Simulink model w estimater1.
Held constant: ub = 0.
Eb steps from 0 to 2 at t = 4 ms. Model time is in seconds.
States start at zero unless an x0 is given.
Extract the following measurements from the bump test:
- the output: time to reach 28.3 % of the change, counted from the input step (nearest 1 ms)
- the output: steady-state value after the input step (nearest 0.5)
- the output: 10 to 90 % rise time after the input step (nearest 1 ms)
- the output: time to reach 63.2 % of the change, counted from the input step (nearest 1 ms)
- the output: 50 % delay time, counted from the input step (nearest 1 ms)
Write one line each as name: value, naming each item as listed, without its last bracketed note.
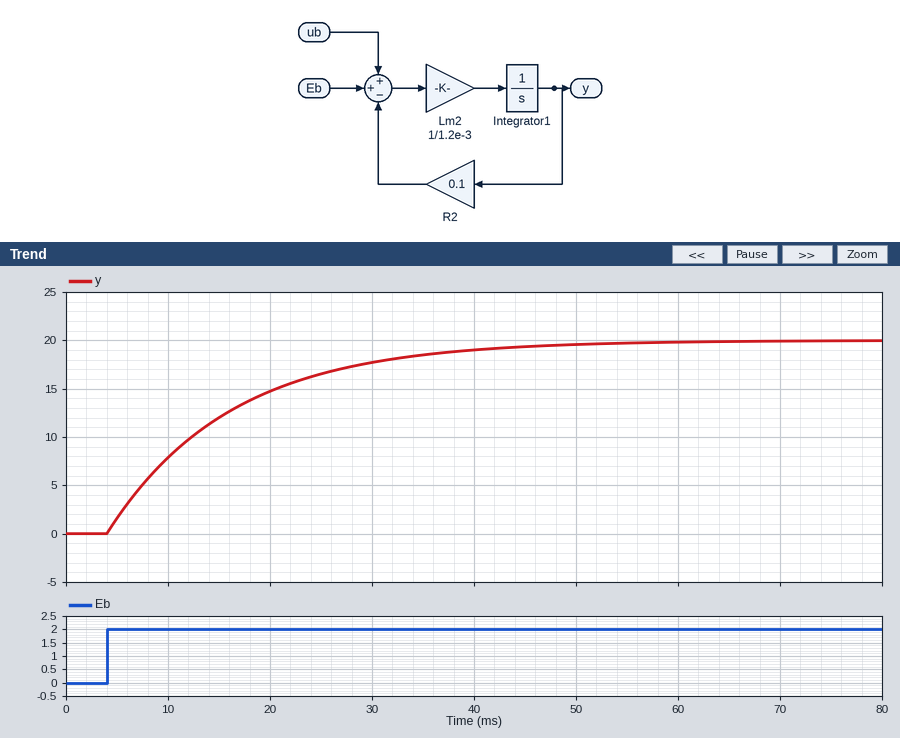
the output: time to reach 28.3 % of the change, counted from the input step: 4 ms
the output: steady-state value after the input step: 20.0
the output: 10 to 90 % rise time after the input step: 26 ms
the output: time to reach 63.2 % of the change, counted from the input step: 12 ms
the output: 50 % delay time, counted from the input step: 8 ms
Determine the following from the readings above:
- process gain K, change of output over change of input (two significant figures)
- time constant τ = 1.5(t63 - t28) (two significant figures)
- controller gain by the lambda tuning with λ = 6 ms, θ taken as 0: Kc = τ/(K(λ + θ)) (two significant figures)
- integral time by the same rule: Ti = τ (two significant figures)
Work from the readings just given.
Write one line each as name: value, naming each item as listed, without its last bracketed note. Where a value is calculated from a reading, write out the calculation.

process gain K, change of output over change of input: (20 - 0) / 2 = 10
time constant τ = 1.5(t63 - t28): 1.5 × (12 - 4) = 12 ms
controller gain by the lambda tuning with λ = 6 ms, θ taken as 0: Kc = τ/(K(λ + θ)): 12 / (10 × (6 + 0)) = 0.20
integral time by the same rule: Ti = τ: 12 ms
